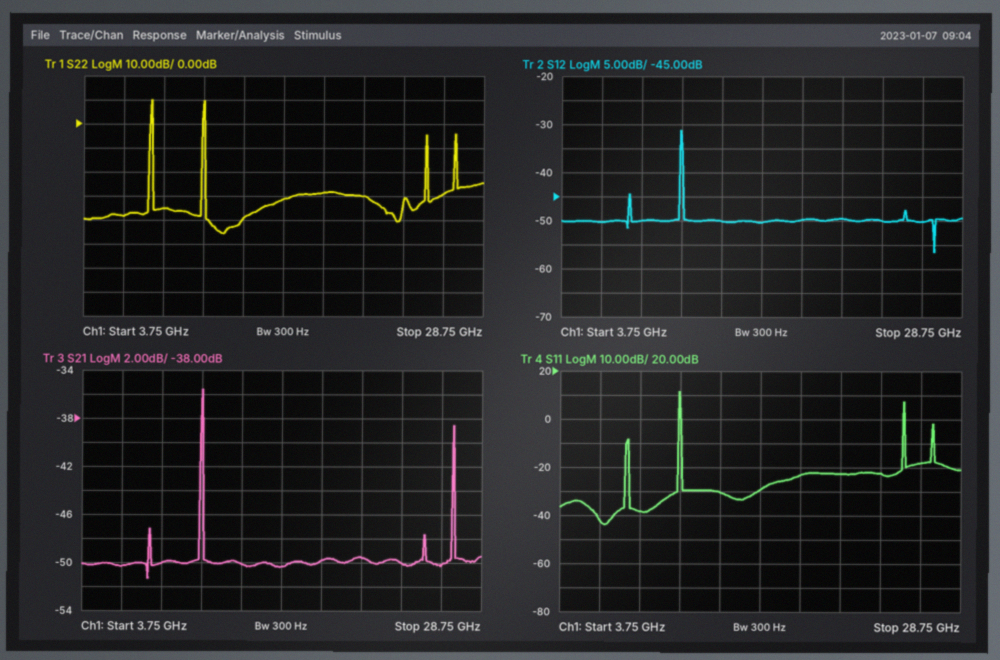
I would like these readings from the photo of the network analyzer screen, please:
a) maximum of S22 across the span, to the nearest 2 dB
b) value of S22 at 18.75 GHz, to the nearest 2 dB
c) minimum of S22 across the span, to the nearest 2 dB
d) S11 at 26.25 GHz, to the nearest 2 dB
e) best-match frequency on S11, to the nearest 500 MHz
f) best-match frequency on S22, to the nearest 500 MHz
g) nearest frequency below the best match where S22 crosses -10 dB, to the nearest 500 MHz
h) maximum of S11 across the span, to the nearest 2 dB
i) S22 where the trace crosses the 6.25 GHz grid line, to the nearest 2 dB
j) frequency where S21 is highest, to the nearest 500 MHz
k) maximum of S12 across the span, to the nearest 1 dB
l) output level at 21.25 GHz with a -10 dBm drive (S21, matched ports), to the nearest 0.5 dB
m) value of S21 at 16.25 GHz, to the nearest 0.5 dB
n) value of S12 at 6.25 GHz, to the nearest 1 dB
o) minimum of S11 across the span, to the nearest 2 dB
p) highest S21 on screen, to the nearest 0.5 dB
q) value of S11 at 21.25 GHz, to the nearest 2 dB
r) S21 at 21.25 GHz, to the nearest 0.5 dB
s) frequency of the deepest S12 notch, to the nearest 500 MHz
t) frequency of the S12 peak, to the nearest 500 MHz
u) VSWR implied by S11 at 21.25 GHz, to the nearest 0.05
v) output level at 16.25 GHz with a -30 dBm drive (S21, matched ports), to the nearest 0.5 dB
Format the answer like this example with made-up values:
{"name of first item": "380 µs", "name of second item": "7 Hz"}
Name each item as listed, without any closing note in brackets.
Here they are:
{"maximum of S22 across the span, to the nearest 2 dB": "10 dB", "value of S22 at 18.75 GHz, to the nearest 2 dB": "-28 dB", "minimum of S22 across the span, to the nearest 2 dB": "-46 dB", "S11 at 26.25 GHz, to the nearest 2 dB": "-18 dB", "best-match frequency on S11, to the nearest 500 MHz": "6.5 GHz", "best-match frequency on S22, to the nearest 500 MHz": "12.5 GHz", "nearest frequency below the best match where S22 crosses -10 dB, to the nearest 500 MHz": "11.5 GHz", "maximum of S11 across the span, to the nearest 2 dB": "12 dB", "S22 where the trace crosses the 6.25 GHz grid line, to the nearest 2 dB": "-38 dB", "frequency where S21 is highest, to the nearest 500 MHz": "11.5 GHz", "maximum of S12 across the span, to the nearest 1 dB": "-31 dB", "output level at 21.25 GHz with a -10 dBm drive (S21, matched ports), to the nearest 0.5 dB": "-59.5 dBm", "value of S21 at 16.25 GHz, to the nearest 0.5 dB": "-50.5 dB", "value of S12 at 6.25 GHz, to the nearest 1 dB": "-50 dB", "minimum of S11 across the span, to the nearest 2 dB": "-44 dB", "highest S21 on screen, to the nearest 0.5 dB": "-35.5 dB", "value of S11 at 21.25 GHz, to the nearest 2 dB": "-22 dB", "S21 at 21.25 GHz, to the nearest 0.5 dB": "-49.5 dB", "frequency of the deepest S12 notch, to the nearest 500 MHz": "27.0 GHz", "frequency of the S12 peak, to the nearest 500 MHz": "11.0 GHz", "VSWR implied by S11 at 21.25 GHz, to the nearest 0.05": "1.15", "output level at 16.25 GHz with a -30 dBm drive (S21, matched ports), to the nearest 0.5 dB": "-80.5 dBm"}
